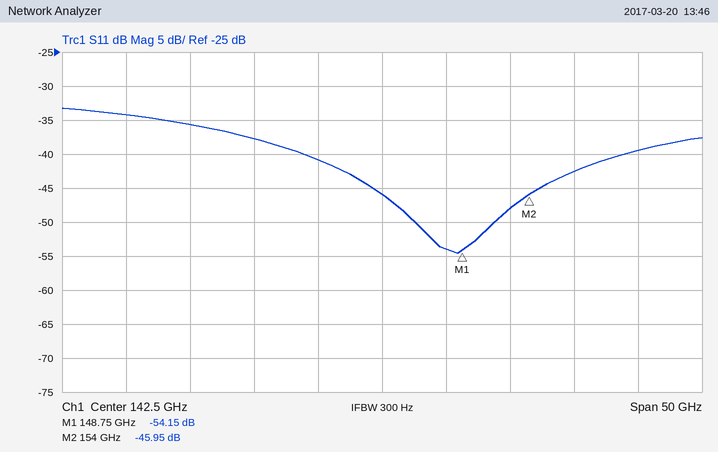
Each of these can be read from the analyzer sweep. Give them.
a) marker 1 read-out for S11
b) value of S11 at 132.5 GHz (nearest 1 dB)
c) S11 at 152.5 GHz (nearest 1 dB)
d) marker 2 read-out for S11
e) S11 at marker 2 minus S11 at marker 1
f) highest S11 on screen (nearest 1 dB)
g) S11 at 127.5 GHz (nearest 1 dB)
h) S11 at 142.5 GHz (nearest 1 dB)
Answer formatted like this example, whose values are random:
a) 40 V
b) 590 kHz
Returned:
a) -54.15 dB
b) -38 dB
c) -48 dB
d) -45.95 dB
e) 8.20 dB
f) -33 dB
g) -36 dB
h) -46 dB
